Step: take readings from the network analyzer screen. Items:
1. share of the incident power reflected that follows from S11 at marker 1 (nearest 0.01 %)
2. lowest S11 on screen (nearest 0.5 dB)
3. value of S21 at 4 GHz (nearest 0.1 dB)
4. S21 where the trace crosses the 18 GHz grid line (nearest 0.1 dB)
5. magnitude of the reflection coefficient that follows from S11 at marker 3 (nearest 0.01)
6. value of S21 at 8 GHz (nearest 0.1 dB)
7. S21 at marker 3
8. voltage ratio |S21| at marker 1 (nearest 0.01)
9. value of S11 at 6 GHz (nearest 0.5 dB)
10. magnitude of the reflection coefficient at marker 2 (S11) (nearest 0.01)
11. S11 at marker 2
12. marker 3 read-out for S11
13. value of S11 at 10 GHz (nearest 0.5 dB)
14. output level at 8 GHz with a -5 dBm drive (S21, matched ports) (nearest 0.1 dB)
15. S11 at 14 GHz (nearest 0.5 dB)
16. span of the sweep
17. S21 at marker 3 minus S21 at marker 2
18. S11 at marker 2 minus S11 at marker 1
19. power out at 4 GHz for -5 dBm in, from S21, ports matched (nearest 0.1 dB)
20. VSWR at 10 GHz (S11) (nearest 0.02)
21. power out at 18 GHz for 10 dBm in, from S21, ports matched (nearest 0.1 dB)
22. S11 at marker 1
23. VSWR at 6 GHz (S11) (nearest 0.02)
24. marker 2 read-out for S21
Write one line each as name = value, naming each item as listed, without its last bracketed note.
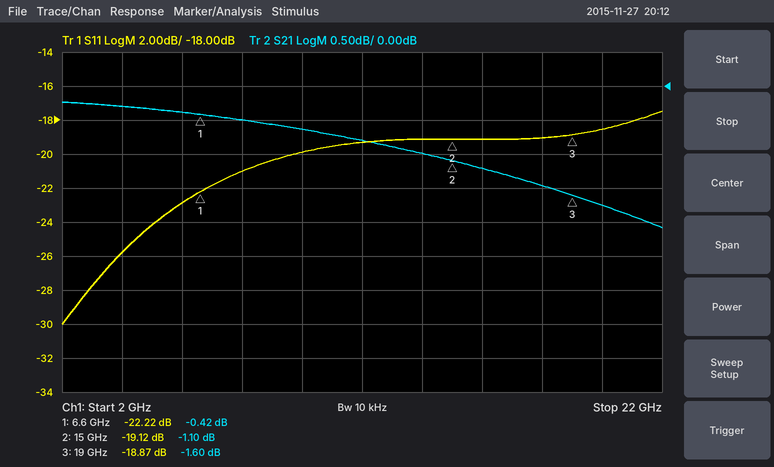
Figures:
share of the incident power reflected that follows from S11 at marker 1 = 0.60 %
lowest S11 on screen = -30.0 dB
value of S21 at 4 GHz = -0.3 dB
S21 where the trace crosses the 18 GHz grid line = -1.5 dB
magnitude of the reflection coefficient that follows from S11 at marker 3 = 0.11
value of S21 at 8 GHz = -0.5 dB
S21 at marker 3 = -1.60 dB
voltage ratio |S21| at marker 1 = 0.95
value of S11 at 6 GHz = -23.0 dB
magnitude of the reflection coefficient at marker 2 (S11) = 0.11
S11 at marker 2 = -19.12 dB
marker 3 read-out for S11 = -18.87 dB
value of S11 at 10 GHz = -20.0 dB
output level at 8 GHz with a -5 dBm drive (S21, matched ports) = -5.5 dBm
S11 at 14 GHz = -19.0 dB
span of the sweep = 20 GHz
S21 at marker 3 minus S21 at marker 2 = -0.50 dB
S11 at marker 2 minus S11 at marker 1 = 3.10 dB
power out at 4 GHz for -5 dBm in, from S21, ports matched = -5.3 dBm
VSWR at 10 GHz (S11) = 1.22
power out at 18 GHz for 10 dBm in, from S21, ports matched = 8.5 dBm
S11 at marker 1 = -22.22 dB
VSWR at 6 GHz (S11) = 1.16
marker 2 read-out for S21 = -1.10 dB
